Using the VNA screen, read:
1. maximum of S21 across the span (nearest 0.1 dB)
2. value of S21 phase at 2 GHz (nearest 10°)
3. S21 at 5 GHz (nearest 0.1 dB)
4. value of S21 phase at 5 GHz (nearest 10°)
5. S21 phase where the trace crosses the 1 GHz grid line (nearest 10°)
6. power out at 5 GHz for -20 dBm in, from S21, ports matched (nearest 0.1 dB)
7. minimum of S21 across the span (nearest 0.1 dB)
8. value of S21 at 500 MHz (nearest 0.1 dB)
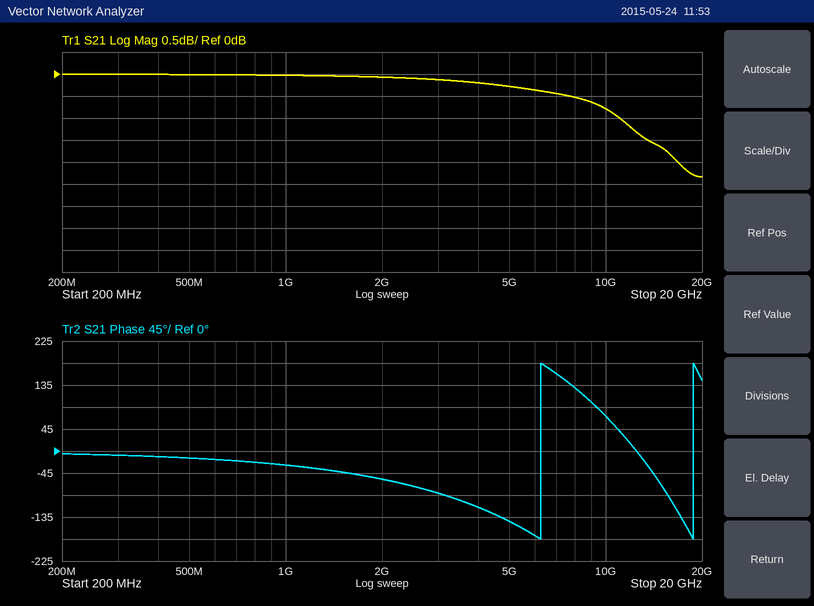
0.0 dB
-60°
-0.3 dB
-140°
-30°
-20.3 dBm
-2.3 dB
0.0 dB
